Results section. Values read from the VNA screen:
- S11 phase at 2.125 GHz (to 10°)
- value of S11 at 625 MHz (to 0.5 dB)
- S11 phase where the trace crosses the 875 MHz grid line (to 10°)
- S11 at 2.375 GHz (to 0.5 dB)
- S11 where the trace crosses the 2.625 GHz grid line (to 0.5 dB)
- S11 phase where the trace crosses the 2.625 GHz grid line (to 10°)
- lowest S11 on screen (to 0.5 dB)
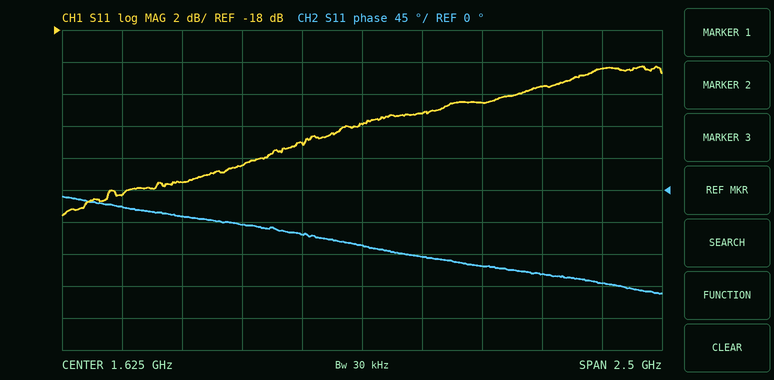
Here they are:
-110°
-28.5 dB
-40°
-21.5 dB
-20.5 dB
-130°
-29.5 dB
